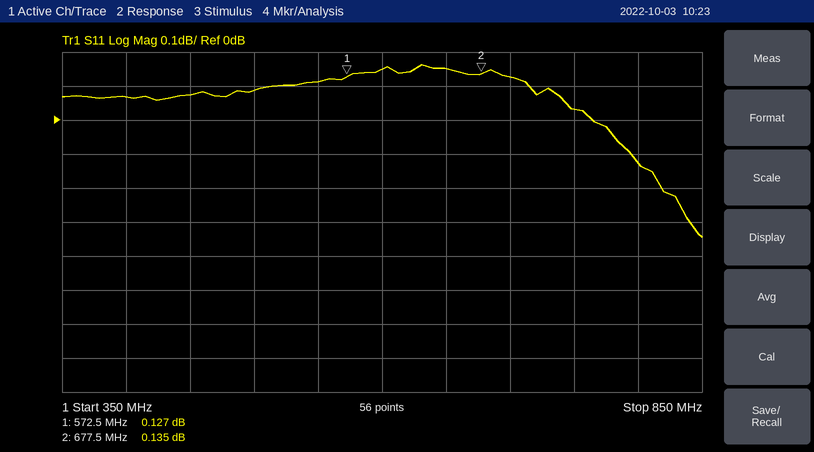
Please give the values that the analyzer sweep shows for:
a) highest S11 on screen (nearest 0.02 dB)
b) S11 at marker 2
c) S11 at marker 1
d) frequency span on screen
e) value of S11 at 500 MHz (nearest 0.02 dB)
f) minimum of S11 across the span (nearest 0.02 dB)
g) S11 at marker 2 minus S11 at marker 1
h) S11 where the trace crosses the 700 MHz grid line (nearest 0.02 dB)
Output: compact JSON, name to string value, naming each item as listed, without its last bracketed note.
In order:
{"highest S11 on screen": "0.16 dB", "S11 at marker 2": "0.135 dB", "S11 at marker 1": "0.127 dB", "frequency span on screen": "500 MHz", "value of S11 at 500 MHz": "0.08 dB", "minimum of S11 across the span": "-0.34 dB", "S11 at marker 2 minus S11 at marker 1": "0.008 dB", "S11 where the trace crosses the 700 MHz grid line": "0.12 dB"}
